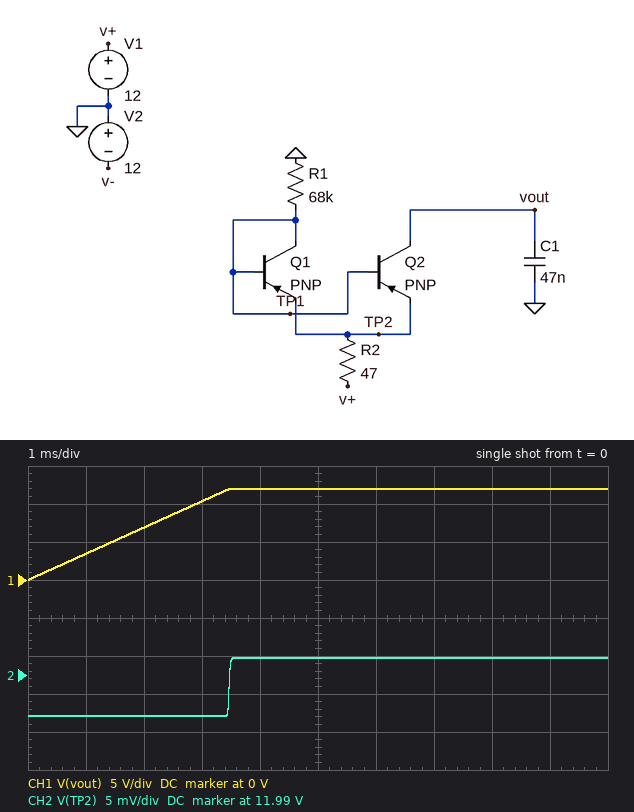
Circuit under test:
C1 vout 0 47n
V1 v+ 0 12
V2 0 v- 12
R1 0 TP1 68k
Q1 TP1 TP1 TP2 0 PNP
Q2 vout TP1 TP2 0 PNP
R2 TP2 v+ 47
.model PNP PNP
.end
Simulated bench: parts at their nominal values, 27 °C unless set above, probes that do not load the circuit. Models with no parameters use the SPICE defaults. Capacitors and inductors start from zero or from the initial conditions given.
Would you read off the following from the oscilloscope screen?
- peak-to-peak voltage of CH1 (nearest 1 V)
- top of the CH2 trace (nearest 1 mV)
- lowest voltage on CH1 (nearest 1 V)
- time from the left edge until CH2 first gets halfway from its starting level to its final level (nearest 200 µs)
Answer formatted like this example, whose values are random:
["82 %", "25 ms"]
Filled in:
["12 V", "11.992 V", "0 V", "3.4 ms"]
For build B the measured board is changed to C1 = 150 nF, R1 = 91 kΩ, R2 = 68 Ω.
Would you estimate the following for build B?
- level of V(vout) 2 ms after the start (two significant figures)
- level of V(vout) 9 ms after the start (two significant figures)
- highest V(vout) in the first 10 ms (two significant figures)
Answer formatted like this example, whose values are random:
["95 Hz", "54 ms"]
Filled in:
["1.6 V", "7.3 V", "8.1 V"]
